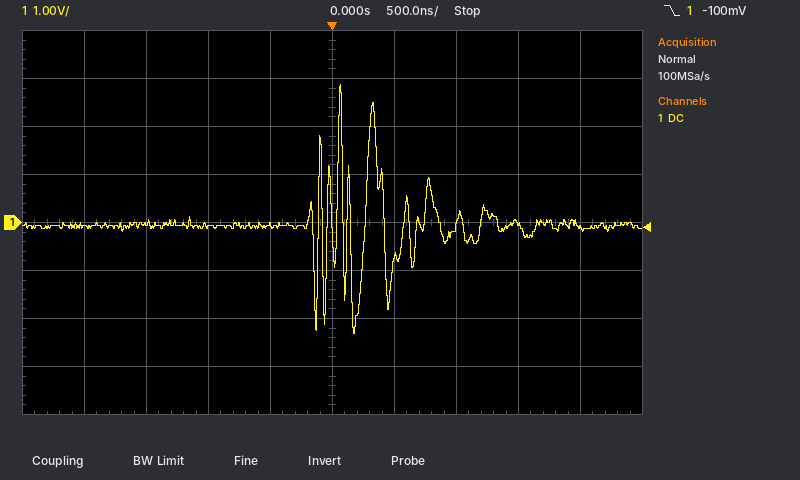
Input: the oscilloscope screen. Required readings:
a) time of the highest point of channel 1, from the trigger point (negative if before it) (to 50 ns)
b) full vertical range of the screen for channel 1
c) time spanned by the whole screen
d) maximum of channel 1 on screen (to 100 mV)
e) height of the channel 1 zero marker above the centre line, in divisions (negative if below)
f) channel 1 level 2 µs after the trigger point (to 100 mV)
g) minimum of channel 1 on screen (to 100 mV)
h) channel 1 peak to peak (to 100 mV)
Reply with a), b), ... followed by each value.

a) +50 ns
b) 8 V
c) 5 µs
d) 2.9 V
e) 0.0 div
f) -100 mV
g) -2.3 V
h) 5.2 V
